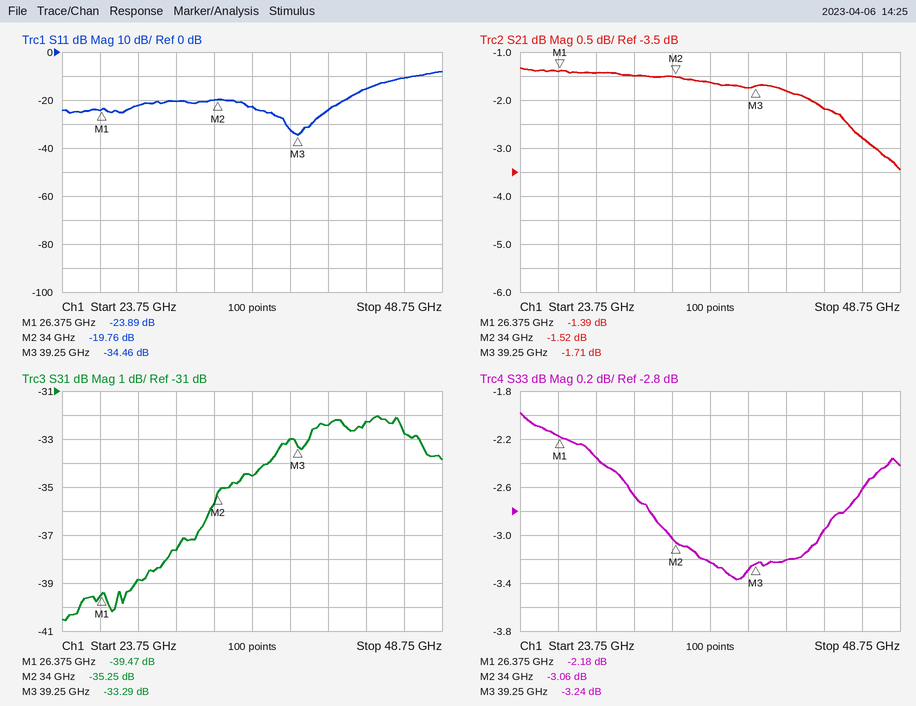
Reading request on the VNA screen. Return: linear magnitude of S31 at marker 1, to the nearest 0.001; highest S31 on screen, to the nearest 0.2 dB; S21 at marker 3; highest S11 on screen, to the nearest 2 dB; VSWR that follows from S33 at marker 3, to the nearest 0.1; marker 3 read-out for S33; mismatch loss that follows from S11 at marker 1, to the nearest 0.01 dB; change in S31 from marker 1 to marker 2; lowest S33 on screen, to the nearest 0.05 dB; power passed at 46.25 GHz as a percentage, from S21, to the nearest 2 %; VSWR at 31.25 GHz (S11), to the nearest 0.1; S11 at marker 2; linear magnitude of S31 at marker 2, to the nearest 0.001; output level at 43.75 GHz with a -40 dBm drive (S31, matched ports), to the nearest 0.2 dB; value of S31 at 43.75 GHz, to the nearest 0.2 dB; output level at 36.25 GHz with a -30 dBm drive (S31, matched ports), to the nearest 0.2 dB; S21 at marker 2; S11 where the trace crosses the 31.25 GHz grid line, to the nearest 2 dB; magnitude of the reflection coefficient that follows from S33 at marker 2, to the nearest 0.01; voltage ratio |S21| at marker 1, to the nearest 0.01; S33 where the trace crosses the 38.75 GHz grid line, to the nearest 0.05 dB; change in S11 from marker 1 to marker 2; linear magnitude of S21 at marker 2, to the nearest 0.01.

0.011
-32.0 dB
-1.71 dB
-8 dB
5.4
-3.24 dB
0.02 dB
4.22 dB
-3.35 dB
52 %
1.2
-19.76 dB
0.017
-72.2 dBm
-32.2 dB
-64.6 dBm
-1.52 dB
-20 dB
0.70
0.85
-3.30 dB
4.13 dB
0.84
